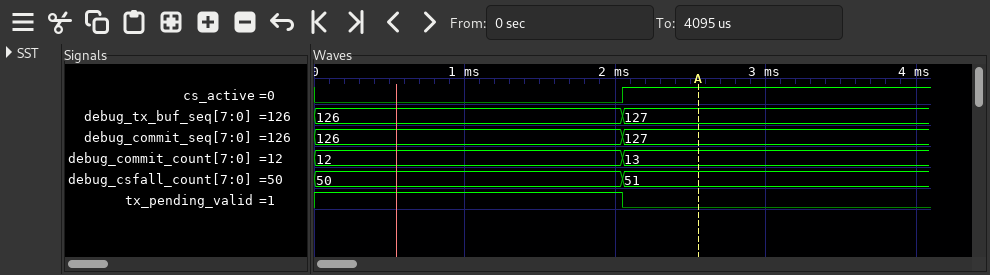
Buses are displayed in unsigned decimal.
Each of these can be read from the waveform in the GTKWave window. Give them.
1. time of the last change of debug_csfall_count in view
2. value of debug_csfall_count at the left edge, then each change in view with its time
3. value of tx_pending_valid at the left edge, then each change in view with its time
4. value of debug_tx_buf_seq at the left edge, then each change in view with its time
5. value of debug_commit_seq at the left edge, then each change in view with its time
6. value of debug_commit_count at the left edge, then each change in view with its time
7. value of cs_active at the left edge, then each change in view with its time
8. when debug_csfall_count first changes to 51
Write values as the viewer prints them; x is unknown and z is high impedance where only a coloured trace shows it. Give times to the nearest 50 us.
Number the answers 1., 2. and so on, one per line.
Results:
1. 2050 us
2. 50, 51 at 2050 us
3. 1, 0 at 2050 us
4. 126, 127 at 2050 us
5. 126, 127 at 2050 us
6. 12, 13 at 2050 us
7. 0, 1 at 2050 us
8. 2050 us
